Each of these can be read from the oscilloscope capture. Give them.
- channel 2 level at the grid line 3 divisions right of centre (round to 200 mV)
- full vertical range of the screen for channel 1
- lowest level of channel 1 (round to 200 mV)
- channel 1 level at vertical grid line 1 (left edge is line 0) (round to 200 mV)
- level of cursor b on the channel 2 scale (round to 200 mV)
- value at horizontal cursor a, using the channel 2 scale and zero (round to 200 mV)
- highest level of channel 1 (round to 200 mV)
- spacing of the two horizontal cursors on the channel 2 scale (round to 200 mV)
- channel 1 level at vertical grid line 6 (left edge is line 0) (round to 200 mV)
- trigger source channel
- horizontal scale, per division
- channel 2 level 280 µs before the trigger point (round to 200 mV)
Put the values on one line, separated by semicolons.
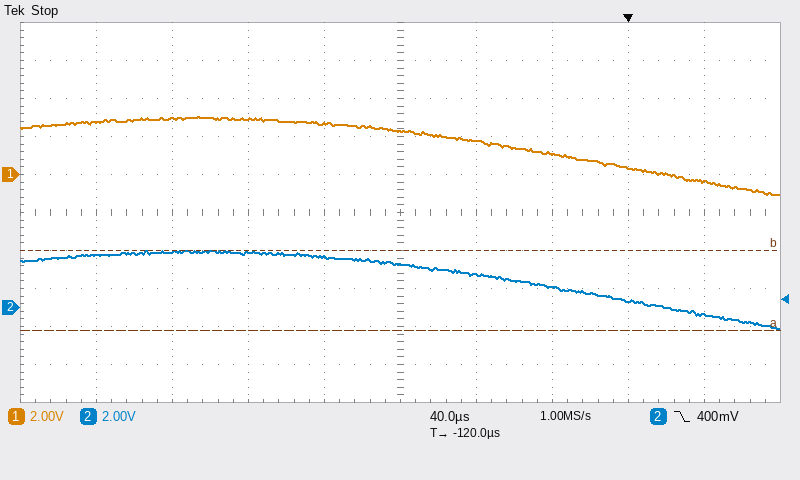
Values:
400 mV; 20 V; -1.0 V; 2.8 V; 3.0 V; -1.2 V; 3.0 V; 4.2 V; 1.8 V; channel 2; 40 µs; 2.8 V
